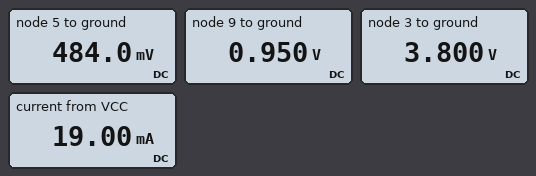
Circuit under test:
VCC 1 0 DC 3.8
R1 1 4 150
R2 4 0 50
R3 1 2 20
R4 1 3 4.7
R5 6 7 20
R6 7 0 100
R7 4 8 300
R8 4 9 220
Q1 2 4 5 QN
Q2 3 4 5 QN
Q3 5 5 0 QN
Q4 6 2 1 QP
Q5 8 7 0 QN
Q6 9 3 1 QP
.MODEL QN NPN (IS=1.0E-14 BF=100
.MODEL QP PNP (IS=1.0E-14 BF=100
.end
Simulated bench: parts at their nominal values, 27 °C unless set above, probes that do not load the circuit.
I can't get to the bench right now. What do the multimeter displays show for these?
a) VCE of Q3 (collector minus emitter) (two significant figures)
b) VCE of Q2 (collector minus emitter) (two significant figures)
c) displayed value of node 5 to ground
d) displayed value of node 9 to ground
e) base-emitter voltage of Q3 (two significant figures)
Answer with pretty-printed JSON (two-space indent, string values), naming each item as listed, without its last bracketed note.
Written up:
{
  "VCE of Q3 (collector minus emitter)": "480 mV",
  "VCE of Q2 (collector minus emitter)": "3.3 V",
  "displayed value of node 5 to ground": "484.0 mV",
  "displayed value of node 9 to ground": "0.950 V",
  "base-emitter voltage of Q3": "480 mV"
}
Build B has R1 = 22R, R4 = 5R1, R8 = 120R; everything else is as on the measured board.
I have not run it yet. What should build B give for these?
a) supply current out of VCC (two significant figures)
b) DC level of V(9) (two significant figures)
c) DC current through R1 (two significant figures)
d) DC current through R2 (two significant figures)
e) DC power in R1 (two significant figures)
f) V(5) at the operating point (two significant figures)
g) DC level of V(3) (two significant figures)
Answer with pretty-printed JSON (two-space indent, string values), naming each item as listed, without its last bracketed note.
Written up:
{
  "supply current out of VCC": "7.2 A",
  "DC level of V(9)": "3.8 V",
  "DC current through R1": "93 mA",
  "DC current through R2": "35 mA",
  "DC power in R1": "190 mW",
  "V(5) at the operating point": "880 mV",
  "DC level of V(3)": "2.9 V"
}
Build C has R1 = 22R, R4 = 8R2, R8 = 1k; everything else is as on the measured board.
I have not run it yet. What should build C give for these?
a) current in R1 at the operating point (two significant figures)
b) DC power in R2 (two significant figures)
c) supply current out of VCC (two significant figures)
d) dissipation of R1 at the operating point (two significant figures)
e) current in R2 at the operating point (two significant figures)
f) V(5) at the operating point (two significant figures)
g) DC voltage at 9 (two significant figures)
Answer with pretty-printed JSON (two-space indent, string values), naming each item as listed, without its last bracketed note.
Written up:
{
  "current in R1 at the operating point": "94 mA",
  "DC power in R2": "60 mW",
  "supply current out of VCC": "5.8 A",
  "dissipation of R1 at the operating point": "190 mW",
  "current in R2 at the operating point": "35 mA",
  "V(5) at the operating point": "880 mV",
  "DC voltage at 9": "3.8 V"
}
